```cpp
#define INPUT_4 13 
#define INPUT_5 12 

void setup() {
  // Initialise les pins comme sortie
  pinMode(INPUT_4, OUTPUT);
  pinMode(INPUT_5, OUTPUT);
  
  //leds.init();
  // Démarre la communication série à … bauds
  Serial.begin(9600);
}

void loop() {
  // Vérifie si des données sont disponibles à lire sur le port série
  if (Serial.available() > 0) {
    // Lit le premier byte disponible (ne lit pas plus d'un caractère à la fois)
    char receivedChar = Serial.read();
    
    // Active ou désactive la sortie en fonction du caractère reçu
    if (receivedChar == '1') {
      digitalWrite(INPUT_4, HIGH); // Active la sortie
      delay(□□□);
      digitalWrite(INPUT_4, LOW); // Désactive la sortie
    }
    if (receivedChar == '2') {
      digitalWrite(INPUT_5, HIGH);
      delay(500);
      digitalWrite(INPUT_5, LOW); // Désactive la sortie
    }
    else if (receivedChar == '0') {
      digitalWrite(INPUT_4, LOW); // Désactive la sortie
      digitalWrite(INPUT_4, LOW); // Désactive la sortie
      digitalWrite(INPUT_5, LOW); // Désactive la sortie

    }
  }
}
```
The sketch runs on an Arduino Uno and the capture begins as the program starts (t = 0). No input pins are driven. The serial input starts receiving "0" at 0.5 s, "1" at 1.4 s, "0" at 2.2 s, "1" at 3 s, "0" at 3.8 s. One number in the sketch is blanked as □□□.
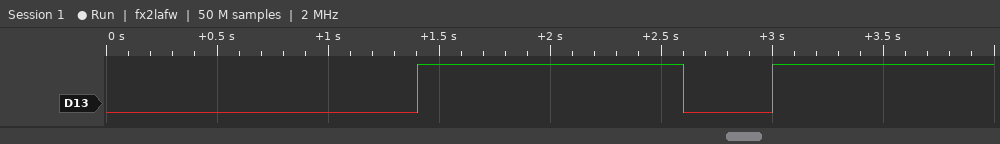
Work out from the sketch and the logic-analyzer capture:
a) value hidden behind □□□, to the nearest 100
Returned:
1200
